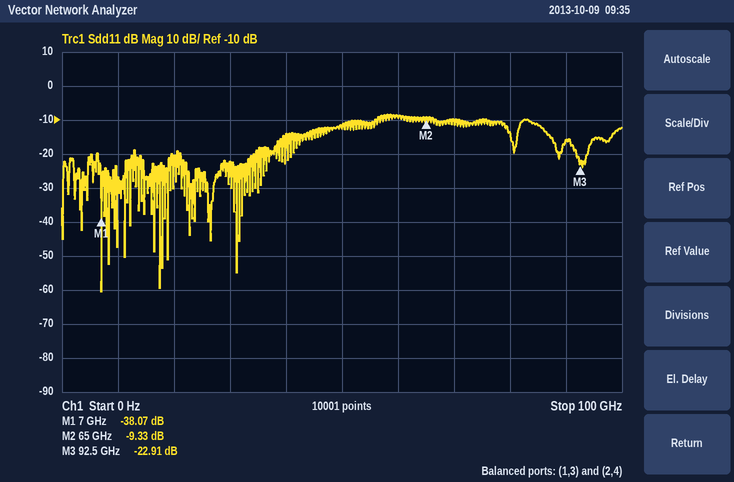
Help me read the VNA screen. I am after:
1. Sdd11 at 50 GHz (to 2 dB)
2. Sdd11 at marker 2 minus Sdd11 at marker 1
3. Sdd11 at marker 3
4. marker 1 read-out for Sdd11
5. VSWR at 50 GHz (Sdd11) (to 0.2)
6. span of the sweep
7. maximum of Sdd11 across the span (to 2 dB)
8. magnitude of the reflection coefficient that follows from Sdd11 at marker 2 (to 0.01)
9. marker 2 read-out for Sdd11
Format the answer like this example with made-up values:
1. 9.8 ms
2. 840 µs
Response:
1. -12 dB
2. 28.74 dB
3. -22.91 dB
4. -38.07 dB
5. 1.6
6. 100 GHz
7. -8 dB
8. 0.34
9. -9.33 dB
